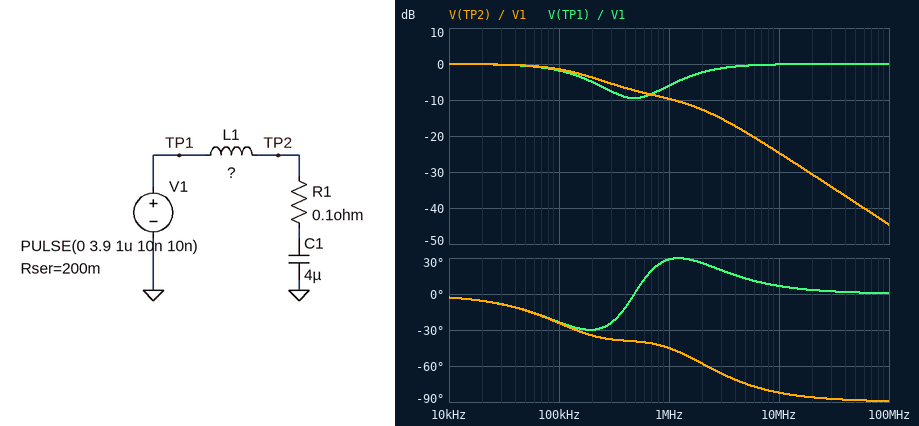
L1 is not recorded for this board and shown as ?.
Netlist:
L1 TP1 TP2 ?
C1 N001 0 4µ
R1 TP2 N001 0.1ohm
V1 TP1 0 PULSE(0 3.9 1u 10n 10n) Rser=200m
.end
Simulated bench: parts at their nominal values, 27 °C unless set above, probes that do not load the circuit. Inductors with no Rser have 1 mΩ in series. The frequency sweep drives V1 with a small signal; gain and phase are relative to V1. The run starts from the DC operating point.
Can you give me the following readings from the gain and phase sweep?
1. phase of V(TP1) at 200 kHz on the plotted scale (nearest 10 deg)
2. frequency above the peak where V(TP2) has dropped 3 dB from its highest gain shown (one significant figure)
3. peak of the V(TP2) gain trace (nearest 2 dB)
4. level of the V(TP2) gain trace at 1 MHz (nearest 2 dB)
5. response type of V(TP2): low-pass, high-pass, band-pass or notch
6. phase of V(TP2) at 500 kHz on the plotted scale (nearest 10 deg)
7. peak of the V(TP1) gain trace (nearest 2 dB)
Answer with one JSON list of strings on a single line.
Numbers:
["-30 deg", "200 kHz", "0 dB", "-10 dB", "low-pass", "-40 deg", "0 dB"]
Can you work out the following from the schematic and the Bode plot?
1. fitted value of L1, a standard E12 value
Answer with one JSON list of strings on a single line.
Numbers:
["27 nH"]
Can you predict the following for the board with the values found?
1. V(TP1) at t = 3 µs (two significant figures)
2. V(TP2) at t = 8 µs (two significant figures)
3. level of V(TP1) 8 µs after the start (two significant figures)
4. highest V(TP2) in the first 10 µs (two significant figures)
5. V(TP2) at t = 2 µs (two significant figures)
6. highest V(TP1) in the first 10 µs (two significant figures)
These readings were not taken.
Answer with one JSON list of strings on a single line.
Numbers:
["3.4 V", "3.9 V", "3.9 V", "3.9 V", "2.8 V", "3.9 V"]
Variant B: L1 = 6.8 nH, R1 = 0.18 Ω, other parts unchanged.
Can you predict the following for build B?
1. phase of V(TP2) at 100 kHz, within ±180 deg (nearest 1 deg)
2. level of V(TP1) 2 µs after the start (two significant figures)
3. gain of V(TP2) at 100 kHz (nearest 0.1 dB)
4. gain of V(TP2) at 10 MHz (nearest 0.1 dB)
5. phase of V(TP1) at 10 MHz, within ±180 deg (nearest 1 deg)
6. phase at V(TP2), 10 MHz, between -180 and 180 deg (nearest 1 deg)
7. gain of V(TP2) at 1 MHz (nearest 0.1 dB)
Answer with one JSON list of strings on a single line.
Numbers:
["-20 deg", "2.8 V", "-2.0 dB", "-10.0 dB", "19 deg", "-49 deg", "-6.3 dB"]
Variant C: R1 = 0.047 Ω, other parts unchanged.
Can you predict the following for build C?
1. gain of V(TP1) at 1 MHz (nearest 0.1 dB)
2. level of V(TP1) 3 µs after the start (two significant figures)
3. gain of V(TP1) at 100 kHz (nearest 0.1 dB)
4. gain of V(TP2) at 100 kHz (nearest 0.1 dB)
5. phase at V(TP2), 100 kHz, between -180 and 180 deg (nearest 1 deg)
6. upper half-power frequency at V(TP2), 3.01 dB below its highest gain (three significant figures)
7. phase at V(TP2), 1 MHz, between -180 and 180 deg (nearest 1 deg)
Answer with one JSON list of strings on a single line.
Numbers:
["-6.1 dB", "3.5 V", "-1.5 dB", "-1.1 dB", "-26 deg", "188 kHz", "-68 deg"]
